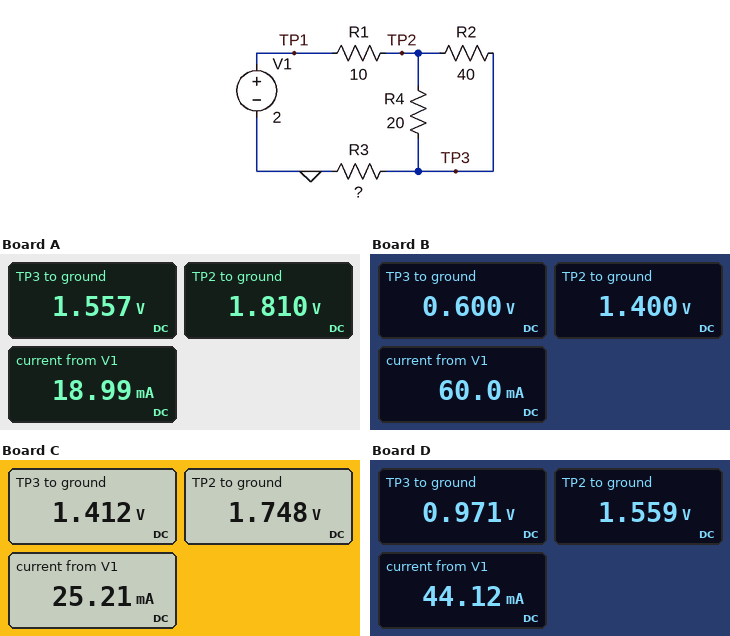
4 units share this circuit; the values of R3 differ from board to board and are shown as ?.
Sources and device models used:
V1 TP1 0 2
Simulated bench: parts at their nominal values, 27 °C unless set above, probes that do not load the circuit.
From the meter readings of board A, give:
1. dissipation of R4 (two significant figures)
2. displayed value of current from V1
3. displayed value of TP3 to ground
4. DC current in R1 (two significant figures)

3.2 mW
18.99 mA
1.557 V
19 mA
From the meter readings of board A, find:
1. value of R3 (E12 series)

82 Ω
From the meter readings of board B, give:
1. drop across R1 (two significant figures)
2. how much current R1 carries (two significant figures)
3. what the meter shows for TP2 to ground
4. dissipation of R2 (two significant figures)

600 mV
60 mA
1.400 V
16 mW
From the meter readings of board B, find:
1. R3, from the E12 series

10 Ω
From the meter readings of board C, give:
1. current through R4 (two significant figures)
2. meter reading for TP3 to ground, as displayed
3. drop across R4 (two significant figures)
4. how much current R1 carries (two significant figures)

17 mA
1.412 V
340 mV
25 mA
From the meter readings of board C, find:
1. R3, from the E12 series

56 Ω
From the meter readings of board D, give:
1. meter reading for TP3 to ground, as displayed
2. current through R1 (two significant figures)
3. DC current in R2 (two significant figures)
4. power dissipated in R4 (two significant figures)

0.971 V
44 mA
15 mA
17 mW
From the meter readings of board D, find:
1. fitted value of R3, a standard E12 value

22 Ω
